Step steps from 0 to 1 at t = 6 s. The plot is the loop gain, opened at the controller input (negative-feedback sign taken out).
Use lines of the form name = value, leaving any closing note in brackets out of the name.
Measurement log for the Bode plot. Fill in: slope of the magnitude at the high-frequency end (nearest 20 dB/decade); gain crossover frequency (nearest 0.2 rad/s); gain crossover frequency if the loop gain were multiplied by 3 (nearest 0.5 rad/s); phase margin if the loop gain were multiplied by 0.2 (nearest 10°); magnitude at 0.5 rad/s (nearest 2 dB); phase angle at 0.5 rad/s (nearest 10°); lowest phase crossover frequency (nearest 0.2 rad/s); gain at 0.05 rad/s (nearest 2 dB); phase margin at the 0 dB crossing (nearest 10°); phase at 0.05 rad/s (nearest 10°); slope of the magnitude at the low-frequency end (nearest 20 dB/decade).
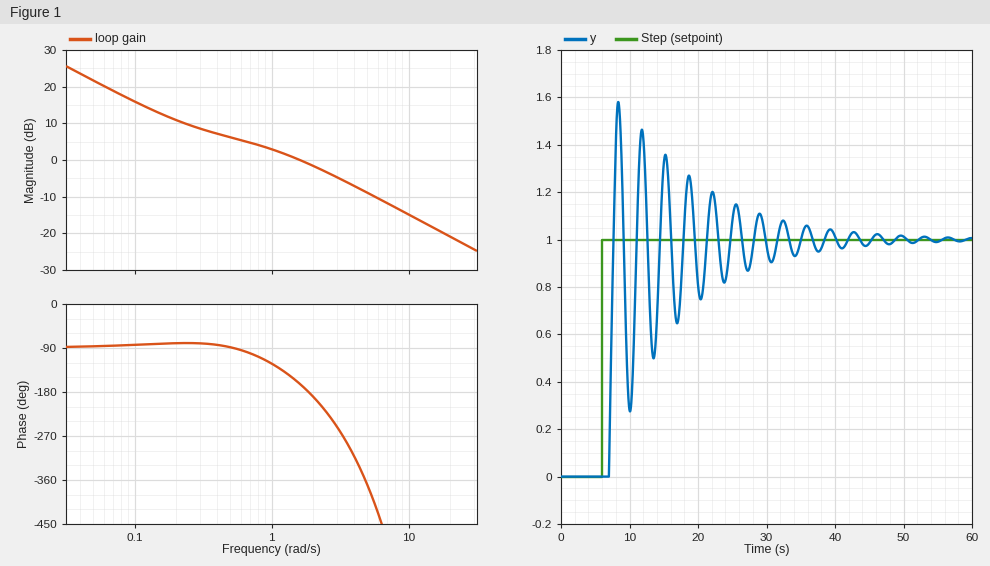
slope of the magnitude at the high-frequency end = -20 dB/decade
gain crossover frequency = 1.6 rad/s
gain crossover frequency if the loop gain were multiplied by 3 = 5.5 rad/s
phase margin if the loop gain were multiplied by 0.2 = 100°
magnitude at 0.5 rad/s = 6 dB
phase angle at 0.5 rad/s = -90°
lowest phase crossover frequency = 1.8 rad/s
gain at 0.05 rad/s = 22 dB
phase margin at the 0 dB crossing = 20°
phase at 0.05 rad/s = -90°
slope of the magnitude at the low-frequency end = -20 dB/decade
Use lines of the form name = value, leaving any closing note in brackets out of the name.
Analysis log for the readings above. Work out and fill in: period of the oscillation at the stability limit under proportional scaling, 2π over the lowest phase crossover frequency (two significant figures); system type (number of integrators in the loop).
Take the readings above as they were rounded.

period of the oscillation at the stability limit under proportional scaling, 2π over the lowest phase crossover frequency = 3.5 s
system type = 1
